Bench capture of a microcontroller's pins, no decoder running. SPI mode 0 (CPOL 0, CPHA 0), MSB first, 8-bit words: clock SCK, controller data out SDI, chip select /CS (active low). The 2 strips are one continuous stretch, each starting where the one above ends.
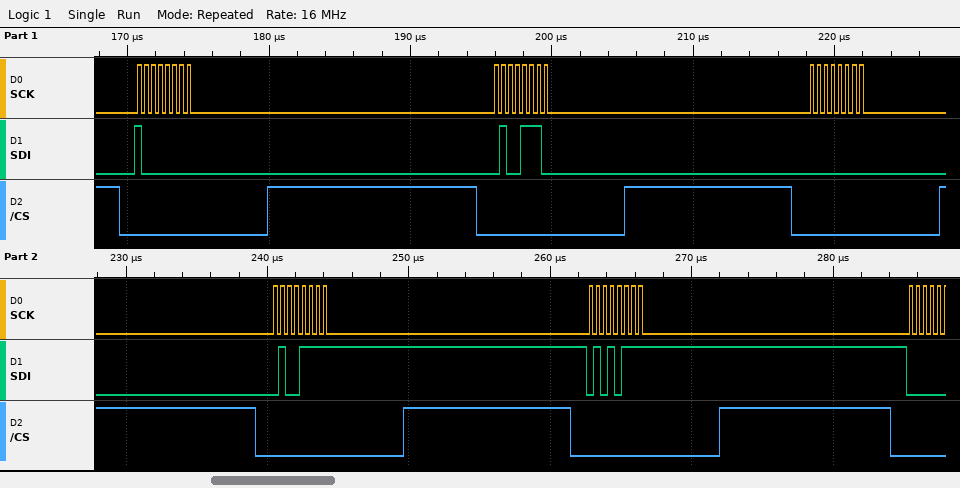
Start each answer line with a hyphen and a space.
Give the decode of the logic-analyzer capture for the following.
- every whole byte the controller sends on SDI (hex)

- 80 4E 00 4F 57
